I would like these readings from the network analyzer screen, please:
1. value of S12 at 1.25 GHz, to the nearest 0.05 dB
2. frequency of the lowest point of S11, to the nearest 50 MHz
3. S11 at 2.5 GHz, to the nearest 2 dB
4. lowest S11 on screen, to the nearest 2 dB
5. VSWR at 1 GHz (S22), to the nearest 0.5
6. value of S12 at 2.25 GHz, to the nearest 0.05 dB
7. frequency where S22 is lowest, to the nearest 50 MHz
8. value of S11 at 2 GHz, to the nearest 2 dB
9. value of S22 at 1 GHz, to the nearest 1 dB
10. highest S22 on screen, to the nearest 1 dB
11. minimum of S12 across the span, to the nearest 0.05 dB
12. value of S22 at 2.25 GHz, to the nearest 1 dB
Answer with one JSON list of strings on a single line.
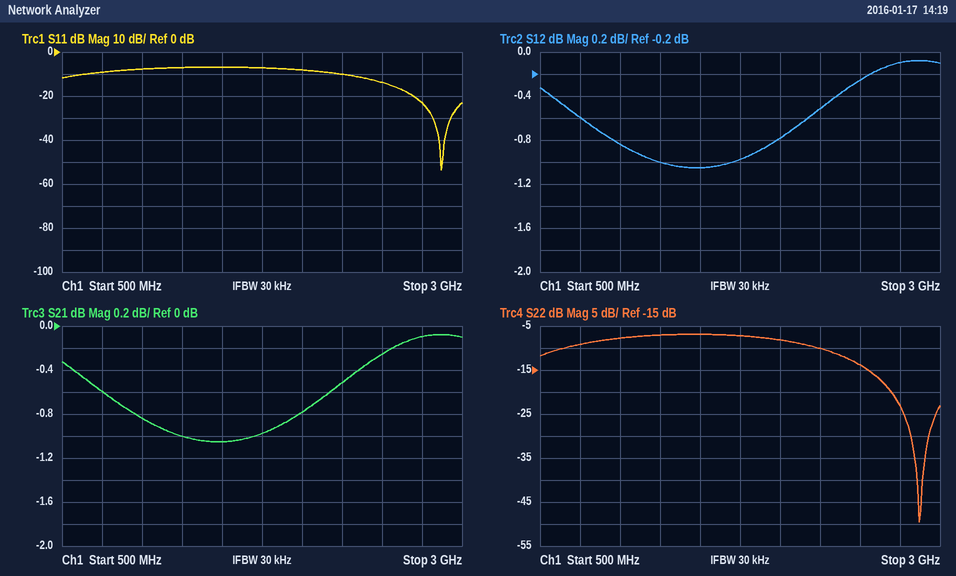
["-1.00 dB", "2.85 GHz", "-14 dB", "-54 dB", "2.5", "-0.50 dB", "2.85 GHz", "-8 dB", "-8 dB", "-7 dB", "-1.05 dB", "-10 dB"]
